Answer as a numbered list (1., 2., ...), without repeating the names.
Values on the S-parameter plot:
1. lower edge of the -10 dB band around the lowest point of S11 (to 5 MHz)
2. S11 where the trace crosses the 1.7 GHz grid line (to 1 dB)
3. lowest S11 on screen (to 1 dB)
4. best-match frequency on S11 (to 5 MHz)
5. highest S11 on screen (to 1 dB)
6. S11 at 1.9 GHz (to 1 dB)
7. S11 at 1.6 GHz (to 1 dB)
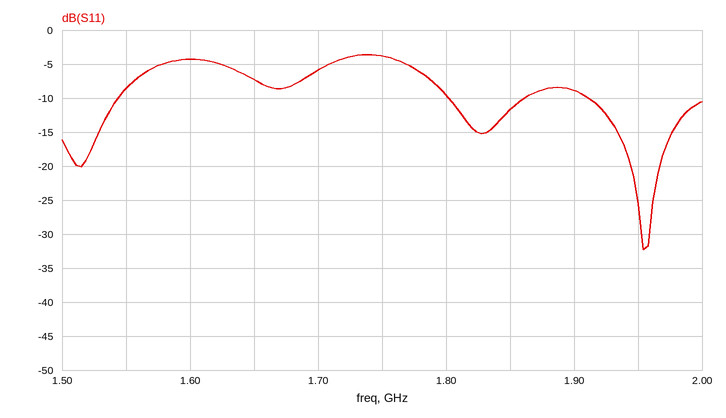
1. 1.910 GHz
2. -6 dB
3. -32 dB
4. 1.955 GHz
5. -4 dB
6. -9 dB
7. -4 dB
